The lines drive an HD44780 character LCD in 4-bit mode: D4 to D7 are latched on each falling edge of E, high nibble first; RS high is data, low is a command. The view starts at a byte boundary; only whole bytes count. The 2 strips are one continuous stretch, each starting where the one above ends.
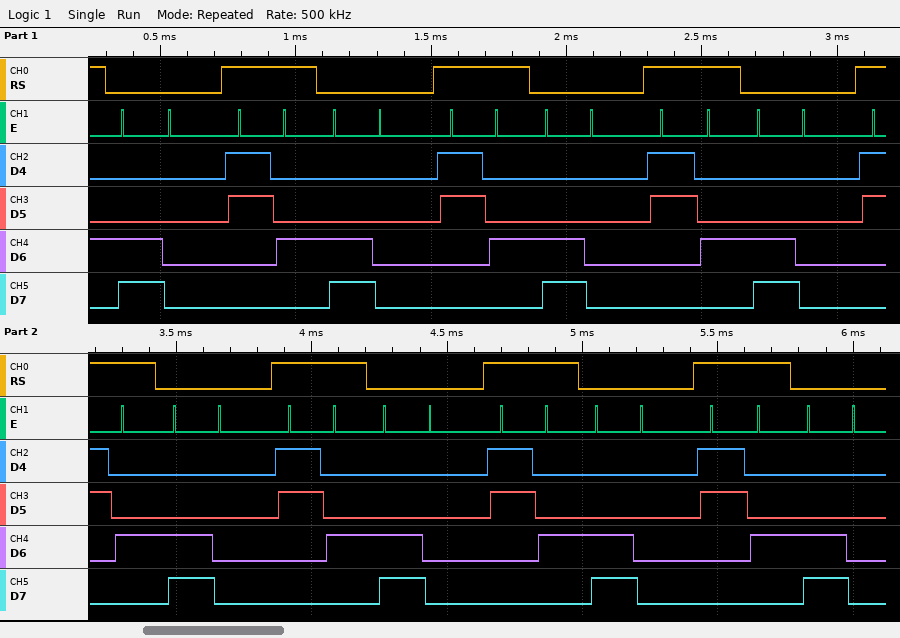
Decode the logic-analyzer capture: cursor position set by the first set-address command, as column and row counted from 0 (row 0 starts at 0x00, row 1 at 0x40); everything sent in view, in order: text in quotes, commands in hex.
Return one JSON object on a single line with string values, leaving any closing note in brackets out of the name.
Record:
{"cursor position set by the first set-address command, as column and row counted from 0": "column 0, row 1", "everything sent in view, in order: text in quotes, commands in hex": "0xC0 \"4\" 0xC0 \"4\" 0xC0 \"4\" 0xC0 \"4\" 0xC0 \"4\" 0xC0 \"4\" 0xC0 \"4\" 0xC0"}
